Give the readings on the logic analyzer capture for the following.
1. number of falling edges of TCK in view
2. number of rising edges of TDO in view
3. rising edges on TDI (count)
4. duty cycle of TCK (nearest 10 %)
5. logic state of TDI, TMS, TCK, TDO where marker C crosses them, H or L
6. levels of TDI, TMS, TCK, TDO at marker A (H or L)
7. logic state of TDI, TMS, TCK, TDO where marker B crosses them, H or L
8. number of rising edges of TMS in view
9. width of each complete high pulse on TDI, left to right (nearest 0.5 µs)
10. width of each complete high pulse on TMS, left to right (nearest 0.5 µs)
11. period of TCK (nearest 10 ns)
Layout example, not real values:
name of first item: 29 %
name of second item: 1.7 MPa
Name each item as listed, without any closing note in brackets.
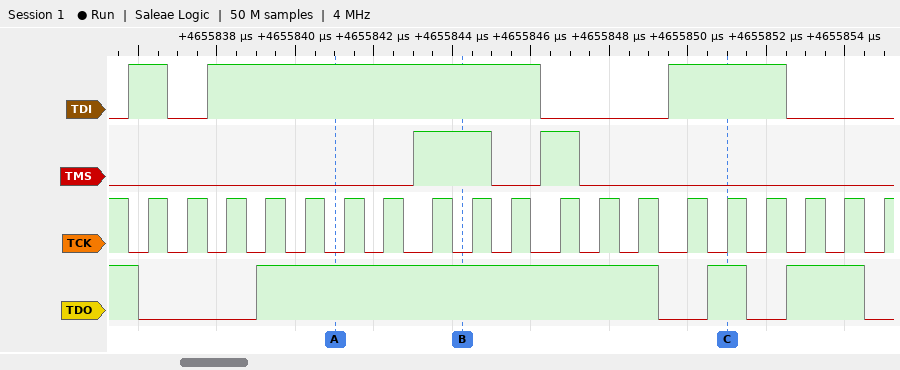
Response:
number of falling edges of TCK in view: 19
number of rising edges of TDO in view: 3
rising edges on TDI: 3
duty cycle of TCK: 50 %
logic state of TDI, TMS, TCK, TDO where marker C crosses them, H or L: TDI=H, TMS=L, TCK=H, TDO=H
levels of TDI, TMS, TCK, TDO at marker A: TDI=H, TMS=L, TCK=L, TDO=H
logic state of TDI, TMS, TCK, TDO where marker B crosses them, H or L: TDI=H, TMS=H, TCK=L, TDO=H
number of rising edges of TMS in view: 2
width of each complete high pulse on TDI, left to right: 1 µs, 8.5 µs, 3 µs
width of each complete high pulse on TMS, left to right: 2 µs, 1 µs
period of TCK: 1040 ns
